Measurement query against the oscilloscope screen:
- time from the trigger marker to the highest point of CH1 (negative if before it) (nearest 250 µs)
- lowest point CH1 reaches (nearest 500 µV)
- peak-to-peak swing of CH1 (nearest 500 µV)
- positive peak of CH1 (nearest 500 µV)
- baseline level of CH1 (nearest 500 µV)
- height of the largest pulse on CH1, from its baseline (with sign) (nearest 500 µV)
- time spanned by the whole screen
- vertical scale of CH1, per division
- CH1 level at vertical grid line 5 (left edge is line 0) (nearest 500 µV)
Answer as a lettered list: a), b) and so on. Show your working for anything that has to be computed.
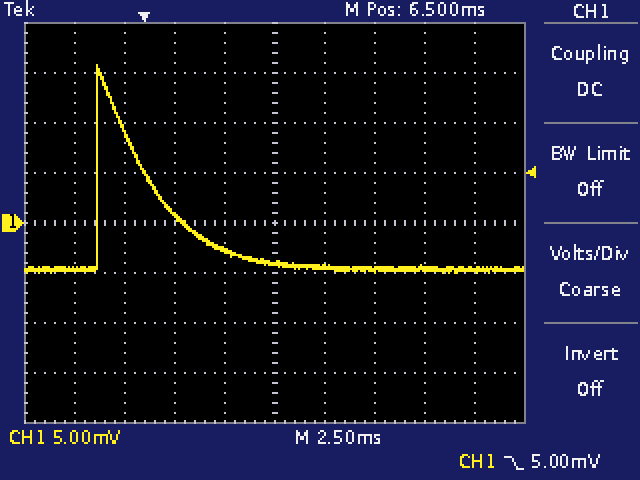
a) -2.25 ms
b) -5.0 mV
c) 16.0 mV − (-5.0 mV) = 21.0 mV
d) 16.0 mV
e) -4.5 mV
f) 16.0 mV − (-4.5 mV) = +20.5 mV
g) 25 ms
h) 5 mV
i) -4.0 mV
